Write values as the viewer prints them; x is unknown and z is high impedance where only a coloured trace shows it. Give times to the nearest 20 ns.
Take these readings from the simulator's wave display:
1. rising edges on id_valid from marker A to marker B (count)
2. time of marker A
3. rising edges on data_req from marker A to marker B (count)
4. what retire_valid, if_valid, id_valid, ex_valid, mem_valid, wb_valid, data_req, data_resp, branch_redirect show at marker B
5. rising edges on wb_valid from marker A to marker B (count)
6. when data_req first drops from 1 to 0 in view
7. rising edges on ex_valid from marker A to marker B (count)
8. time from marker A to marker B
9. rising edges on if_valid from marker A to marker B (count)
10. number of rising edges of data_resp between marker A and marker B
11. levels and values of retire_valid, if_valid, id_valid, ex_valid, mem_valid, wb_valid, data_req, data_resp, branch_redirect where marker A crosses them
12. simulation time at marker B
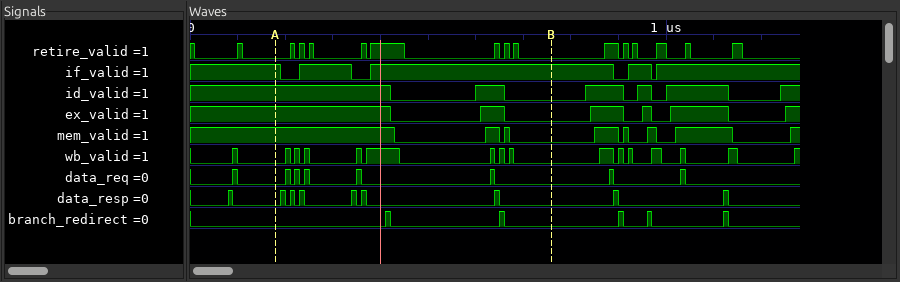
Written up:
1
180 ns
5
retire_valid=0, if_valid=1, id_valid=0, ex_valid=0, mem_valid=0, wb_valid=0, data_req=0, data_resp=0, branch_redirect=0
8
100 ns
1
580 ns
2
6
retire_valid=0, if_valid=1, id_valid=1, ex_valid=1, mem_valid=1, wb_valid=0, data_req=0, data_resp=0, branch_redirect=0
760 ns
